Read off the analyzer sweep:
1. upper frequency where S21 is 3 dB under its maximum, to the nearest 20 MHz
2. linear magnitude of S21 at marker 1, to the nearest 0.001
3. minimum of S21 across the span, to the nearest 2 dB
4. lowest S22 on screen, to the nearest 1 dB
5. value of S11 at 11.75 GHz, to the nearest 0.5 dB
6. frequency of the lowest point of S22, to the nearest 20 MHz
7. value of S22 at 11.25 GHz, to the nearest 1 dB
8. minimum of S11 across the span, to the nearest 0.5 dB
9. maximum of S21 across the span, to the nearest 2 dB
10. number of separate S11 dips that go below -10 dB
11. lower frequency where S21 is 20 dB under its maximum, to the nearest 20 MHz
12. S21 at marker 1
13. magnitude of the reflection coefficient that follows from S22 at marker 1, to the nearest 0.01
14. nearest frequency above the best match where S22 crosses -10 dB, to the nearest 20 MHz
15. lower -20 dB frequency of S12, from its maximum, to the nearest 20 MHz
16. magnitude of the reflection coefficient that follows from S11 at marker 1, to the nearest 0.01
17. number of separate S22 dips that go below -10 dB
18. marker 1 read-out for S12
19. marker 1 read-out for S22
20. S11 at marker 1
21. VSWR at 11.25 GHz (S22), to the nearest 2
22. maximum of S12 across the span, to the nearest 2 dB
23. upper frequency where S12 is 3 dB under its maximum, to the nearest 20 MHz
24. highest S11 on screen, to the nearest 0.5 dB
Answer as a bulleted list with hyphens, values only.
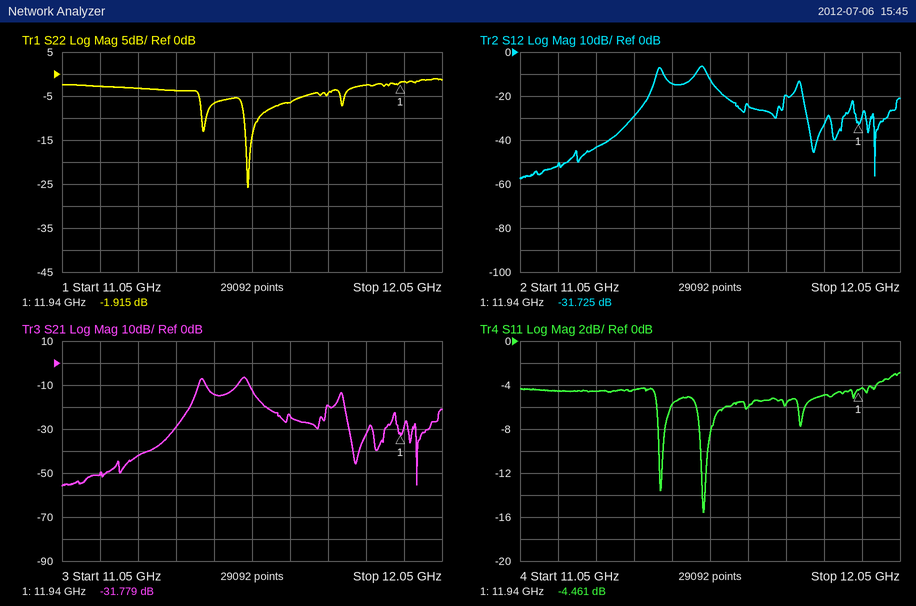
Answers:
- 11.54 GHz
- 0.026
- -56 dB
- -26 dB
- -5.5 dB
- 11.54 GHz
- -3 dB
- -15.5 dB
- -6 dB
- 2
- 11.36 GHz
- -31.779 dB
- 0.80
- 11.56 GHz
- 11.36 GHz
- 0.60
- 2
- -31.725 dB
- -1.915 dB
- -4.461 dB
- 6
- -6 dB
- 11.54 GHz
- -3.0 dB
